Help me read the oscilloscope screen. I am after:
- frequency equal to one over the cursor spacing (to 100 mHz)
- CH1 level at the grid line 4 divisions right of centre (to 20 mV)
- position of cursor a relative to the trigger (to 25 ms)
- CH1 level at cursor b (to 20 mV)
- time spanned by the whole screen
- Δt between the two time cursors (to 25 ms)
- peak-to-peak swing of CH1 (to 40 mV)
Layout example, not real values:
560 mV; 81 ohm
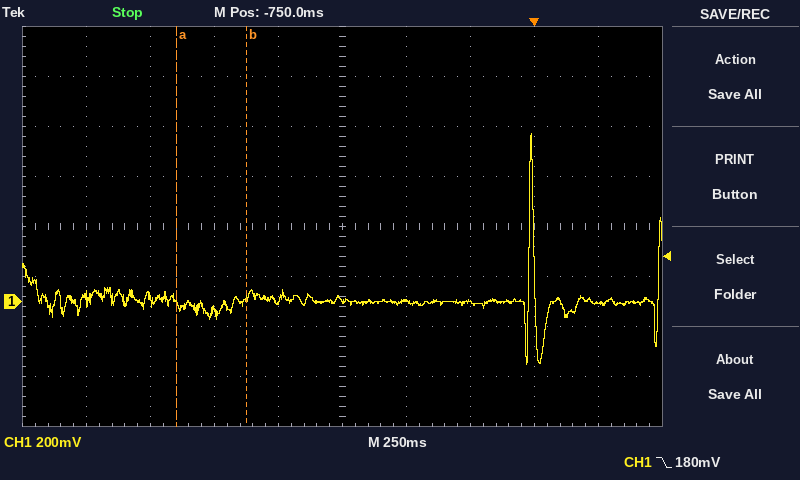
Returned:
3.6 Hz; 0 mV; -1.400 s; 20 mV; 2.5 s; 275 ms; 920 mV
